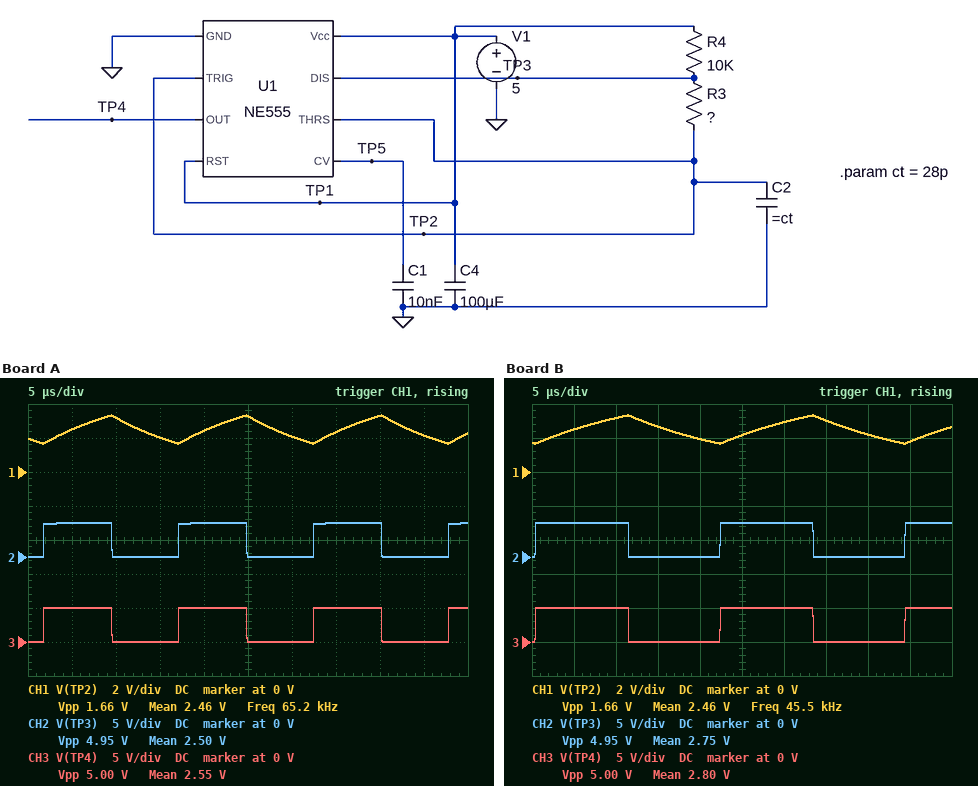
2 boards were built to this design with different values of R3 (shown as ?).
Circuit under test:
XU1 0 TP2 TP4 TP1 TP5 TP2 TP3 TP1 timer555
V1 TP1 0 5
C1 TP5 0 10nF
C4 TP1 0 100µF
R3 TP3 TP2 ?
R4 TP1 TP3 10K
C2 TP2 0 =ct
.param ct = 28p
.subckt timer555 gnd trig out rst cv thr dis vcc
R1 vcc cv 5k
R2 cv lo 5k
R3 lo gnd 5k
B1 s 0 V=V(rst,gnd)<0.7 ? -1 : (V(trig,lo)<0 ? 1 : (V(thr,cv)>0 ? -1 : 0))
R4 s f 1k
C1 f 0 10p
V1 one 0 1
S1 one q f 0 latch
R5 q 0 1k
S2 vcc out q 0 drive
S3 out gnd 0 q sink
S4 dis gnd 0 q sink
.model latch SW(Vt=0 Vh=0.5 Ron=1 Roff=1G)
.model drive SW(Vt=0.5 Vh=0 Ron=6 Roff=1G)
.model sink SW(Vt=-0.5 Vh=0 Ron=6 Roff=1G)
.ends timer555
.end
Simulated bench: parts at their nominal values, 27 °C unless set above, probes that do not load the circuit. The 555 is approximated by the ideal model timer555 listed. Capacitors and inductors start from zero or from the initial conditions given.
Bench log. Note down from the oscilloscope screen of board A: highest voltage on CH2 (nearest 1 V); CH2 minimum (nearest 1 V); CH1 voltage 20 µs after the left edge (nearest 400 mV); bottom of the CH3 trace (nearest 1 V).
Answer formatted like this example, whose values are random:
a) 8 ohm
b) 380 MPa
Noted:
a) 5 V
b) 0 V
c) 2.4 V
d) 0 V
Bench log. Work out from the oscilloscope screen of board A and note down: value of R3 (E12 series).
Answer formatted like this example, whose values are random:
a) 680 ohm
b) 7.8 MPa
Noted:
a) 390 kΩ
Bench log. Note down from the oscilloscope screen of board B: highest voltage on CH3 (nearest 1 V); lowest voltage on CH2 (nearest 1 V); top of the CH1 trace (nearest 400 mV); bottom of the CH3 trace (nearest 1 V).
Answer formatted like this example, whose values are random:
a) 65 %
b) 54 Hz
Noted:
a) 5 V
b) 0 V
c) 3.2 V
d) 0 V
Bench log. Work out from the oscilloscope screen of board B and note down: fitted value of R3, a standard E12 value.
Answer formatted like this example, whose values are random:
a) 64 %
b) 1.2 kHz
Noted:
a) 560 kΩ
